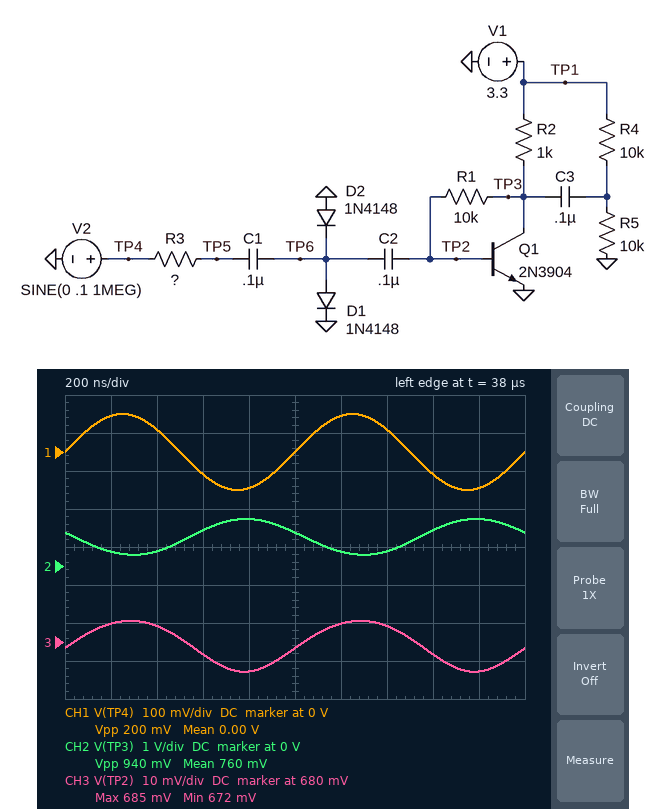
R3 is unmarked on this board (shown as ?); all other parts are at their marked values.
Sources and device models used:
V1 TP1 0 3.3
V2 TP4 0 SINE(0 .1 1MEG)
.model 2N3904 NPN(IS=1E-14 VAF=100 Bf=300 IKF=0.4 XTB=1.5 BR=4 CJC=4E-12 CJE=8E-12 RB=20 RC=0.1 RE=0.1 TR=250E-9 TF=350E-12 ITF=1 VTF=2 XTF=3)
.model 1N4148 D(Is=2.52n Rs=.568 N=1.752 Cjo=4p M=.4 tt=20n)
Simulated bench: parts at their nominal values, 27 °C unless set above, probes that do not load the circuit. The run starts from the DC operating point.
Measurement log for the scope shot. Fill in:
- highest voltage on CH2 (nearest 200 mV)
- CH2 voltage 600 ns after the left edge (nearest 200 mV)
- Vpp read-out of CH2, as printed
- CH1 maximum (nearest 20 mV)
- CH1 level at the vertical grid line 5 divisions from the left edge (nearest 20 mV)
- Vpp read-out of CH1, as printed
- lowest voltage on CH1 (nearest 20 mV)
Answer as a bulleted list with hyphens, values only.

- 1.2 V
- 1.0 V
- 940 mV
- 100 mV
- 0 V
- 200 mV
- -100 mV
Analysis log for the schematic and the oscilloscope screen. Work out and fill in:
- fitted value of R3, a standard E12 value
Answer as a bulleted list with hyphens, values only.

- 1.8 kΩ
